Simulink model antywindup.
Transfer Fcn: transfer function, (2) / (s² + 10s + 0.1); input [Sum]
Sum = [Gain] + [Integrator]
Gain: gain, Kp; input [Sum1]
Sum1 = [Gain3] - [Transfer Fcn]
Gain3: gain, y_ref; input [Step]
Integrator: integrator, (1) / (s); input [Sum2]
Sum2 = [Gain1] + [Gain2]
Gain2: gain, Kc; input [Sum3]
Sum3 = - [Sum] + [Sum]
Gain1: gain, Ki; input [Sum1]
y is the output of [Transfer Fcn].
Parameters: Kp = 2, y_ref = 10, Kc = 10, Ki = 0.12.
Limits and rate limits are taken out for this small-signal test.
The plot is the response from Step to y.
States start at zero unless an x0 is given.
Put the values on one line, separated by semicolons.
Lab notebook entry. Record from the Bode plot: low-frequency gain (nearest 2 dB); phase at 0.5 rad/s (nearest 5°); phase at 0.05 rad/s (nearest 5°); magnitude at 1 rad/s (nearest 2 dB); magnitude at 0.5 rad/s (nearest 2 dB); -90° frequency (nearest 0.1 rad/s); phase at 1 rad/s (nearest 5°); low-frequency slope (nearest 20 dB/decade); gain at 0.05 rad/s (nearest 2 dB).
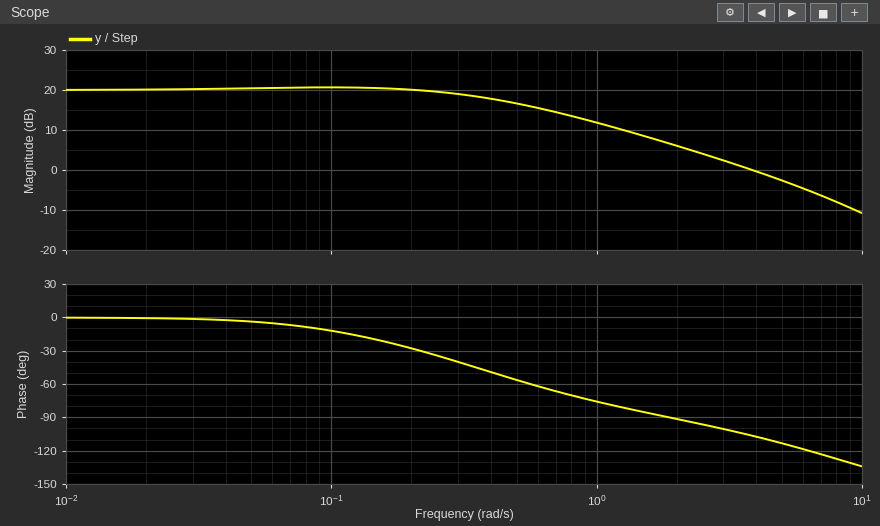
20 dB; -55°; -5°; 12 dB; 16 dB; 1.9 rad/s; -75°; 0 dB/decade; 20 dB
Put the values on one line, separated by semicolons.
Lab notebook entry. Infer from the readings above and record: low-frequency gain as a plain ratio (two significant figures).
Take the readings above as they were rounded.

10
